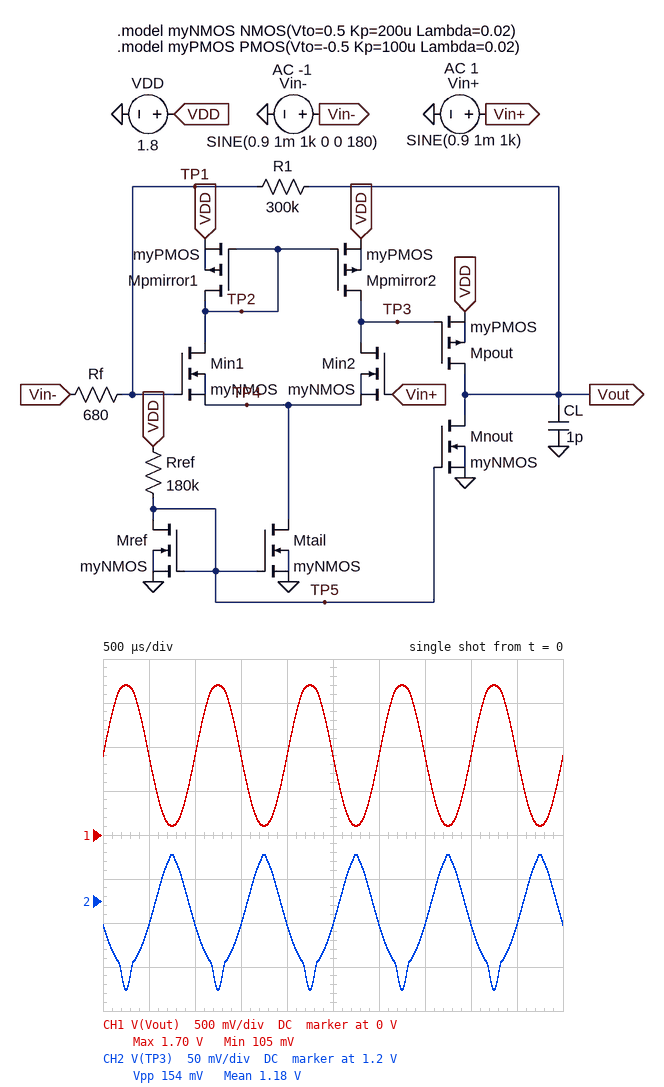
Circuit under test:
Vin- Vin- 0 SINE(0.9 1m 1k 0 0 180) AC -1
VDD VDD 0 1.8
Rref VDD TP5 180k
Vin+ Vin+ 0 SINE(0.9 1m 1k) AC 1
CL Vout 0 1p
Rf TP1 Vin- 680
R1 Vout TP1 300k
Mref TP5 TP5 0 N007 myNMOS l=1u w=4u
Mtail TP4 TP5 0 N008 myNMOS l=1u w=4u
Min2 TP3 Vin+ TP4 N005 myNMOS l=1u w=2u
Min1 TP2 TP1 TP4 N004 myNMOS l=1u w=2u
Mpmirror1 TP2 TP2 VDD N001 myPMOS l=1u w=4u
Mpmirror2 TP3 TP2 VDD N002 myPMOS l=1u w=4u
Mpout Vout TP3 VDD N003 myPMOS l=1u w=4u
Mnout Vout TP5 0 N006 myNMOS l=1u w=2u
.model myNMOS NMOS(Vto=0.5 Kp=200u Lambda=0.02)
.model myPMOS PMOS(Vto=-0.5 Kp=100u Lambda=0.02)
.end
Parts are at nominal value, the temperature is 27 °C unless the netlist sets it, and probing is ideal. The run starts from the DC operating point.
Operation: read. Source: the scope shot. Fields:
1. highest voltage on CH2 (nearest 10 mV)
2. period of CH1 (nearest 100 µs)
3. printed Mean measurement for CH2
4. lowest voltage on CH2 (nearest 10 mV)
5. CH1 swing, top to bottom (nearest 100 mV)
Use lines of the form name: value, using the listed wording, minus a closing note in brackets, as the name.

highest voltage on CH2: 1.25 V
period of CH1: 1.0 ms
printed Mean measurement for CH2: 1.18 V
lowest voltage on CH2: 1.10 V
CH1 swing, top to bottom: 1.6 V
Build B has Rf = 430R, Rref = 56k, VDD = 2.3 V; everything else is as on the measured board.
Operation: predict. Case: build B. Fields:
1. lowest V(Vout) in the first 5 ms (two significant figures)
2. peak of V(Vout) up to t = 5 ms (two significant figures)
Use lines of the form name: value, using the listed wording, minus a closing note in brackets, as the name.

lowest V(Vout) in the first 5 ms: 42 mV
peak of V(Vout) up to t = 5 ms: 2.1 V
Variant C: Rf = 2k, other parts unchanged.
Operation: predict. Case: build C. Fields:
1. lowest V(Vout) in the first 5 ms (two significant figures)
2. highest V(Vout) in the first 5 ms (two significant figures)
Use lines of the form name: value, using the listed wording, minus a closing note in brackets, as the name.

lowest V(Vout) in the first 5 ms: 610 mV
highest V(Vout) in the first 5 ms: 1.2 V
